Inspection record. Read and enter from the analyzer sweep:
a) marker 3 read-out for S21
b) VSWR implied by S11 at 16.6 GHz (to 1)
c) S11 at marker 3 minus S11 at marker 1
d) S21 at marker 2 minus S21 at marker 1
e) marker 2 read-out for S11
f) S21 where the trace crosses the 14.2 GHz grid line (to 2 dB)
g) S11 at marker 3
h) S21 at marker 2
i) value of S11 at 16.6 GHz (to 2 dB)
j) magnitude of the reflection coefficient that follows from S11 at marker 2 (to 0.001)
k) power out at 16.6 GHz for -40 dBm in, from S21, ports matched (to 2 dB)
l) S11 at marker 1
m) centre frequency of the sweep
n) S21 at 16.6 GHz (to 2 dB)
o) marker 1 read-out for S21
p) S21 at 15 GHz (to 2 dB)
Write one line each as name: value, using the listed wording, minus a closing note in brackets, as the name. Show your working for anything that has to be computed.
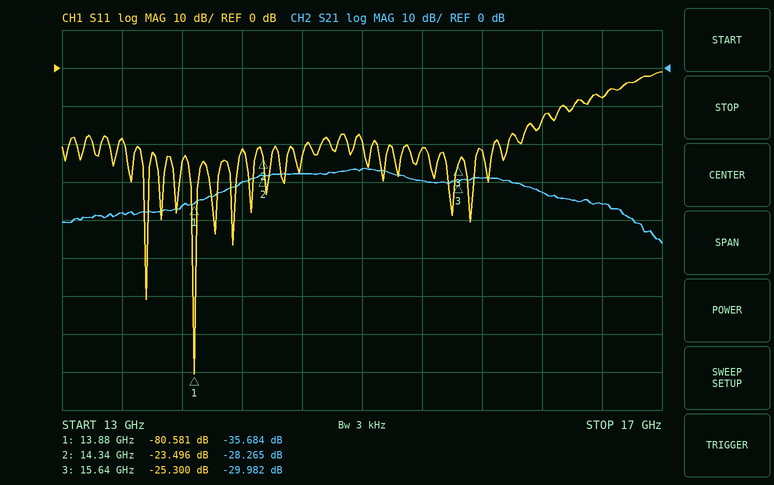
marker 3 read-out for S21: -29.982 dB
VSWR implied by S11 at 16.6 GHz: |Γ| = 10^(-8/20) = 0.3981; VSWR = (1 + 0.3981)/(1 − 0.3981) ≈ 2
S11 at marker 3 minus S11 at marker 1: -25.3 − (-80.581) = 55.281 dB
S21 at marker 2 minus S21 at marker 1: -28.265 − (-35.684) = 7.419 dB
marker 2 read-out for S11: -23.496 dB
S21 where the trace crosses the 14.2 GHz grid line: -30 dB
S11 at marker 3: -25.300 dB
S21 at marker 2: -28.265 dB
value of S11 at 16.6 GHz: -8 dB
magnitude of the reflection coefficient that follows from S11 at marker 2: 10^(-23.496/20) ≈ 0.067
power out at 16.6 GHz for -40 dBm in, from S21, ports matched: -40 dBm + (-36 dB) = -76 dBm
S11 at marker 1: -80.581 dB
centre frequency of the sweep: 15 GHz
S21 at 16.6 GHz: -36 dB
marker 1 read-out for S21: -35.684 dB
S21 at 15 GHz: -26 dB
